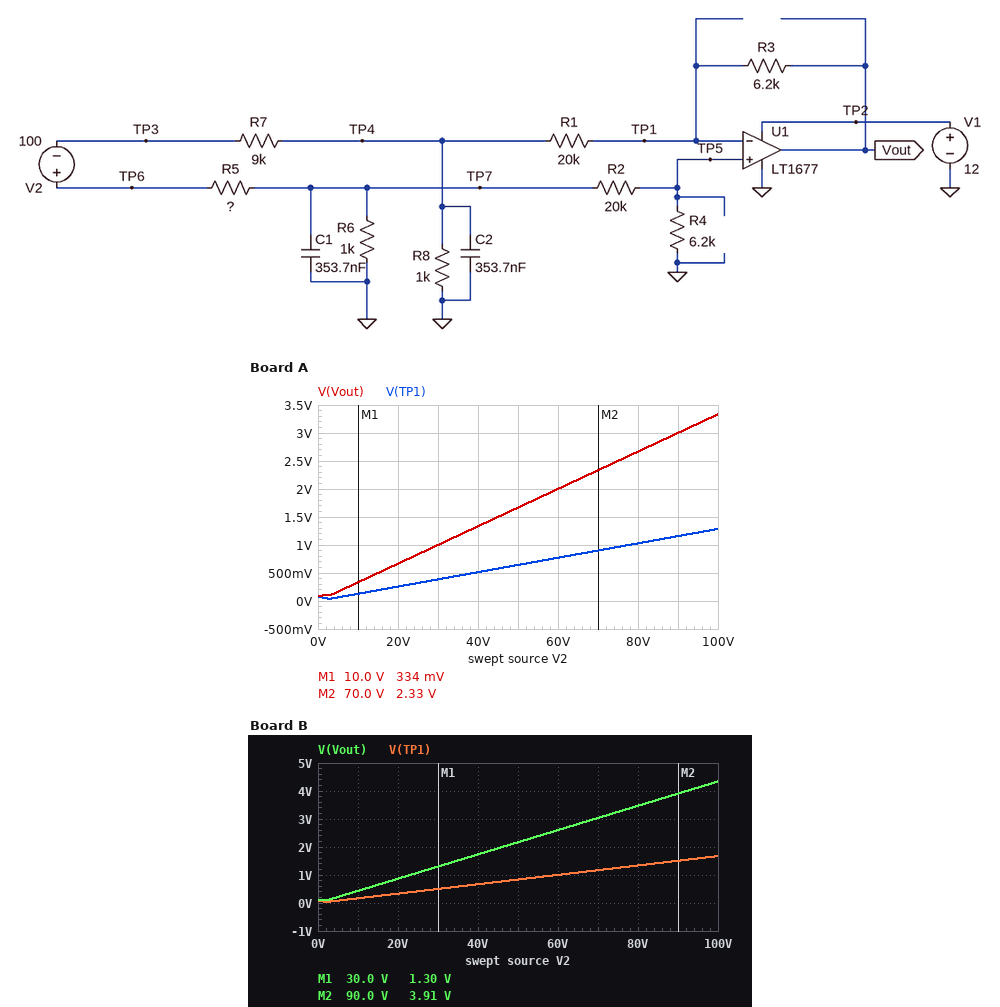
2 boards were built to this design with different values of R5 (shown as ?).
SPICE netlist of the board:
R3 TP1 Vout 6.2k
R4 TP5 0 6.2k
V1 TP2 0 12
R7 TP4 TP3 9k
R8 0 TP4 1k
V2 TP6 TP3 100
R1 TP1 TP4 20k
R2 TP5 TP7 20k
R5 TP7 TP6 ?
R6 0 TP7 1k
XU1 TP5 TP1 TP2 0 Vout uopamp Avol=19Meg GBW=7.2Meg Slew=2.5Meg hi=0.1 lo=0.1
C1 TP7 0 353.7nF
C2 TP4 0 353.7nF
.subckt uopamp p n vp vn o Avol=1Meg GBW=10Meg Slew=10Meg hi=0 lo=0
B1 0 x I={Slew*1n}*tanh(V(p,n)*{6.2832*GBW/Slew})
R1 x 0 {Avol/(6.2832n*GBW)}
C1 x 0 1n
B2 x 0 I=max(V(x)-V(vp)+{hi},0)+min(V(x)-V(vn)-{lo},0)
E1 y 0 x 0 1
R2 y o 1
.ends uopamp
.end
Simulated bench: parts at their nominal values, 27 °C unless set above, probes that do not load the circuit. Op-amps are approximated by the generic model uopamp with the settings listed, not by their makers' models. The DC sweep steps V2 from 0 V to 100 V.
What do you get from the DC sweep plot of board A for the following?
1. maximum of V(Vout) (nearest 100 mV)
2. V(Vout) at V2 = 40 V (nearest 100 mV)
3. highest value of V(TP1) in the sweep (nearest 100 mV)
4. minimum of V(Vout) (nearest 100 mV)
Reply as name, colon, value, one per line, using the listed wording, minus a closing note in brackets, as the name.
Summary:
maximum of V(Vout): 3.3 V
V(Vout) at V2 = 40 V: 1.3 V
highest value of V(TP1) in the sweep: 1.3 V
minimum of V(Vout): 100 mV
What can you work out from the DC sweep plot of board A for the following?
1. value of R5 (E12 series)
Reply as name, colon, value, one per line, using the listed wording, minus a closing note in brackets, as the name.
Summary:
value of R5: 6.8 kΩ
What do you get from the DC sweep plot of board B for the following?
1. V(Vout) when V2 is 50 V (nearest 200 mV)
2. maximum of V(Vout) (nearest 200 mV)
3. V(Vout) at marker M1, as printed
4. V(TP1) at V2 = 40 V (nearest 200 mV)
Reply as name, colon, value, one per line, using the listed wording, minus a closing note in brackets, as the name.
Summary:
V(Vout) when V2 is 50 V: 2.2 V
maximum of V(Vout): 4.4 V
V(Vout) at marker M1, as printed: 1.30 V
V(TP1) at V2 = 40 V: 600 mV
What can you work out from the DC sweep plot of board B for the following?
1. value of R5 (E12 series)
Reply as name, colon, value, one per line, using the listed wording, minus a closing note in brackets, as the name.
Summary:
value of R5: 2.7 kΩ
